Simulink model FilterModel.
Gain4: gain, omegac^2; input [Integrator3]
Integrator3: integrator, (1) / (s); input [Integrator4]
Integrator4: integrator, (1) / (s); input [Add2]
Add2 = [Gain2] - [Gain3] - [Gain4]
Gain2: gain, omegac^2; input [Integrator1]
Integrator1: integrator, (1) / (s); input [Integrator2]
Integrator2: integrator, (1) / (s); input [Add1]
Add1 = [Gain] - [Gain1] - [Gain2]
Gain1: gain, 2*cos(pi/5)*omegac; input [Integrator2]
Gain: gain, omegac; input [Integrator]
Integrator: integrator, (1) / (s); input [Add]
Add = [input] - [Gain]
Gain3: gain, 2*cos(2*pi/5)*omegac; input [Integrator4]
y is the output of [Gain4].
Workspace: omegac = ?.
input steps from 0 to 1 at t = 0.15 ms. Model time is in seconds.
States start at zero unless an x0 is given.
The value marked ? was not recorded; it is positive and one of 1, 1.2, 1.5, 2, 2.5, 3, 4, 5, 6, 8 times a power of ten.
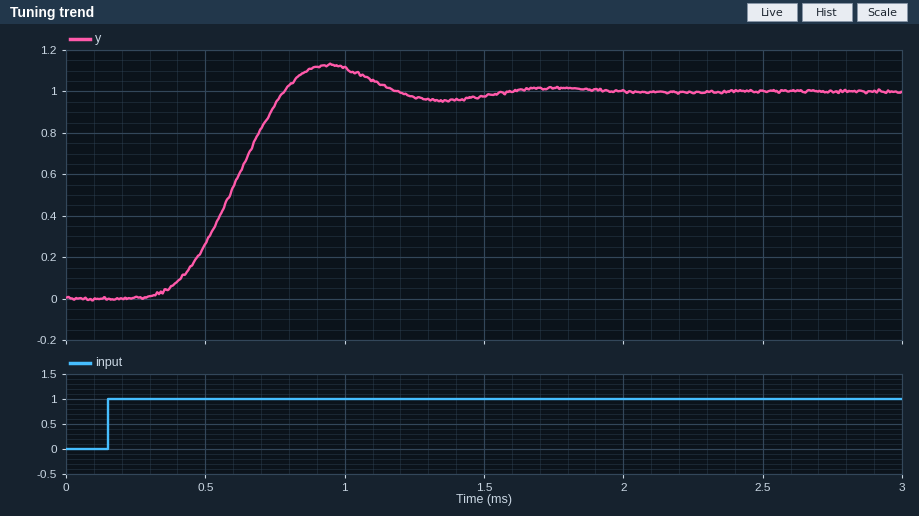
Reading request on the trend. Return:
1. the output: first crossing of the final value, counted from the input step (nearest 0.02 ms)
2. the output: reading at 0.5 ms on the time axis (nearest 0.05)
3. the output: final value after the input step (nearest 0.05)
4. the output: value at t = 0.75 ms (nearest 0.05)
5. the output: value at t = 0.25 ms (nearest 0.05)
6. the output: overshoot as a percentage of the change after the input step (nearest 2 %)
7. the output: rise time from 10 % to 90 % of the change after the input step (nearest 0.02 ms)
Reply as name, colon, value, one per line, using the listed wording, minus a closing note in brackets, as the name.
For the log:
the output: first crossing of the final value, counted from the input step: 0.64 ms
the output: reading at 0.5 ms on the time axis: 0.25
the output: final value after the input step: 1.00
the output: value at t = 0.75 ms: 0.95
the output: value at t = 0.25 ms: 0.00
the output: overshoot as a percentage of the change after the input step: 12 %
the output: rise time from 10 % to 90 % of the change after the input step: 0.32 ms
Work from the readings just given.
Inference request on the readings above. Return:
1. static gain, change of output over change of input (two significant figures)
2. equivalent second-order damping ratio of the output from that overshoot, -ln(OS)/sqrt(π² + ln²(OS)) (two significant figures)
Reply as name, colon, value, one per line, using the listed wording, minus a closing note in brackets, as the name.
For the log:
static gain, change of output over change of input: 1.0
equivalent second-order damping ratio of the output from that overshoot, -ln(OS)/sqrt(π² + ln²(OS)): 0.56
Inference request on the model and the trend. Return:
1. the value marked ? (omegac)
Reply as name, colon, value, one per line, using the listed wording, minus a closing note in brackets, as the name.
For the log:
the value marked ?: 8000
